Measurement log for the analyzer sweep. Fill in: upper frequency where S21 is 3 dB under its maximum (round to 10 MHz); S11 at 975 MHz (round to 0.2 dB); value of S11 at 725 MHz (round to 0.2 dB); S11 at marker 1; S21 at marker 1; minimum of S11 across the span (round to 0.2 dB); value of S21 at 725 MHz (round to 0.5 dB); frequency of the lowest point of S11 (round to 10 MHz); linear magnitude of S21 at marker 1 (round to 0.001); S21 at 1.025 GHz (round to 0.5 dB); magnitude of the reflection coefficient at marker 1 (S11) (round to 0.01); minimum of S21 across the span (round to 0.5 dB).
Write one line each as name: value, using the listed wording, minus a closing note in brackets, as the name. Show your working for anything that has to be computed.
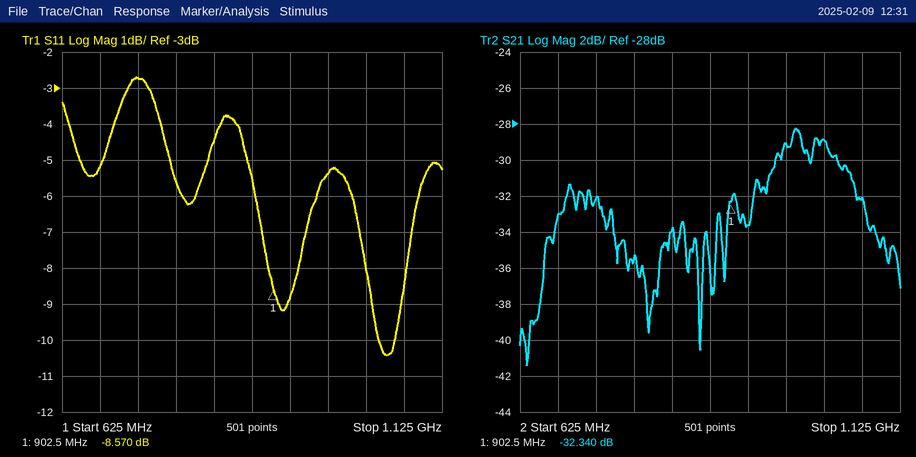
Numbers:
upper frequency where S21 is 3 dB under its maximum: 1.06 GHz
S11 at 975 MHz: -5.4 dB
value of S11 at 725 MHz: -2.8 dB
S11 at marker 1: -8.570 dB
S21 at marker 1: -32.340 dB
minimum of S11 across the span: -10.4 dB
value of S21 at 725 MHz: -32.0 dB
frequency of the lowest point of S11: 1.05 GHz
linear magnitude of S21 at marker 1: 10^(-32.34/20) ≈ 0.024
S21 at 1.025 GHz: -29.0 dB
magnitude of the reflection coefficient at marker 1 (S11): 10^(-8.57/20) ≈ 0.37
minimum of S21 across the span: -41.5 dB
